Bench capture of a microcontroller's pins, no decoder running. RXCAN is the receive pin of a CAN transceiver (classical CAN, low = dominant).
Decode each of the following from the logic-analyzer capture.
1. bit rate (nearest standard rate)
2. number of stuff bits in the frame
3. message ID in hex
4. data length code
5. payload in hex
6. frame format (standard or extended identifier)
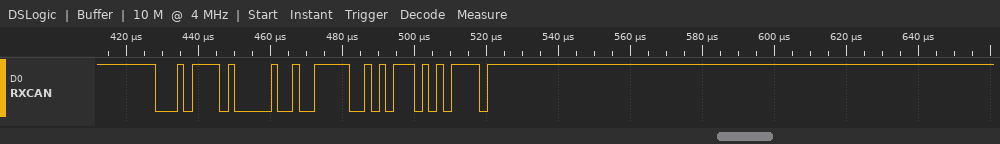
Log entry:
500 kbit/s
2
0x17A
1
3E
standard
